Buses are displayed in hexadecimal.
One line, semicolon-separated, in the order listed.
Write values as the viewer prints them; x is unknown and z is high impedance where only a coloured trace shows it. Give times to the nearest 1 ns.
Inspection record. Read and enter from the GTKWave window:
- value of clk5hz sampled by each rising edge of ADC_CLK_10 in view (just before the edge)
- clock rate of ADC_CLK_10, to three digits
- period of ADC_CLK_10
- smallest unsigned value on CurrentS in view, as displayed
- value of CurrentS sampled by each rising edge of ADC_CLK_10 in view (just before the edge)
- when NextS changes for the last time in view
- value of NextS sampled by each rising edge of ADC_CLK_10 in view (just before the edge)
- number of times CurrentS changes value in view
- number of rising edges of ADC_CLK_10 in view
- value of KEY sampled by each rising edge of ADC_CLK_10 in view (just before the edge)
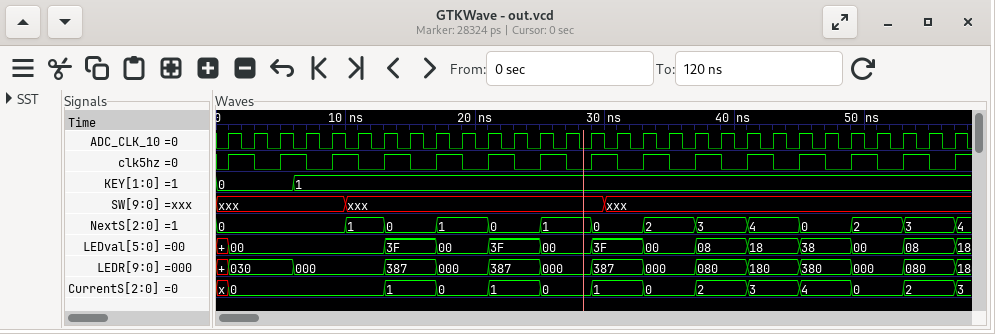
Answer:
0 1 0 1 0 1 0 1 0 1 0 1 0 1 0 1 0 1 0 1 0 1 0 1 0 1 0 1 0; 500 MHz; 2 ns; 0; x, 0, 0, 0, 0, 0, 0, 1, 1, 0, 0, 1, 1, 0, 0, 1, 1, 0, 0, 2, 2, 3, 3, 4, 4, 0, 0, 2, 2; 57 ns; 0, 0, 0, 0, 0, 1, 1, 0, 0, 1, 1, 0, 0, 1, 1, 0, 0, 2, 2, 3, 3, 4, 4, 0, 0, 2, 2, 3, 3; 13; 29; 0, 0, 0, 1, 1, 1, 1, 1, 1, 1, 1, 1, 1, 1, 1, 1, 1, 1, 1, 1, 1, 1, 1, 1, 1, 1, 1, 1, 1
